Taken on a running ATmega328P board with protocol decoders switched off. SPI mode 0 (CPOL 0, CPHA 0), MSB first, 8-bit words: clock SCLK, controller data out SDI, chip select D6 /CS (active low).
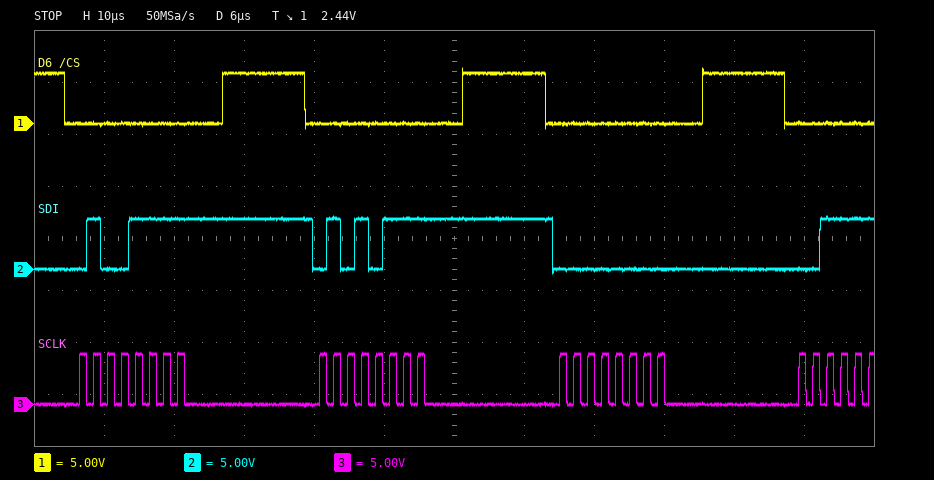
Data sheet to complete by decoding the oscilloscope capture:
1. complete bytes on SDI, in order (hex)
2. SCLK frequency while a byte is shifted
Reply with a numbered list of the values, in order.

1. 4F 57 00
2. 500 kHz
